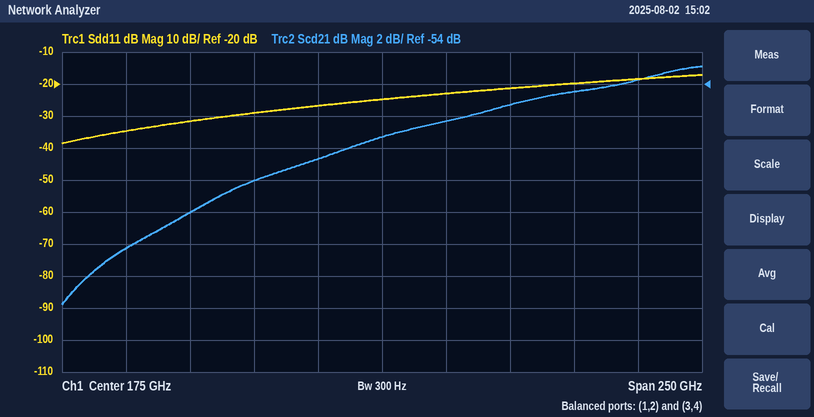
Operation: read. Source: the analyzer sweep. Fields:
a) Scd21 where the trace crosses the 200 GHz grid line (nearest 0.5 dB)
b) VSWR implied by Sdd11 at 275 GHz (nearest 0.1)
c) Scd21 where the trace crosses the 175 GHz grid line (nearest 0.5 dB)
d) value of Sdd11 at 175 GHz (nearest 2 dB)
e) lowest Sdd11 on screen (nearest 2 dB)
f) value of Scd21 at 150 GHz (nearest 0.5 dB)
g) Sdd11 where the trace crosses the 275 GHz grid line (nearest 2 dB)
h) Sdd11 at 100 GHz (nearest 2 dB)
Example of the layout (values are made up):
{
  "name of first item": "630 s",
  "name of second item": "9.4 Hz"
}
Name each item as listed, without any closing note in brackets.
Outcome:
{
  "Scd21 where the trace crosses the 200 GHz grid line": "-56.5 dB",
  "VSWR implied by Sdd11 at 275 GHz": "1.3",
  "Scd21 where the trace crosses the 175 GHz grid line": "-57.5 dB",
  "value of Sdd11 at 175 GHz": "-24 dB",
  "lowest Sdd11 on screen": "-38 dB",
  "value of Scd21 at 150 GHz": "-58.5 dB",
  "Sdd11 where the trace crosses the 275 GHz grid line": "-18 dB",
  "Sdd11 at 100 GHz": "-32 dB"
}
